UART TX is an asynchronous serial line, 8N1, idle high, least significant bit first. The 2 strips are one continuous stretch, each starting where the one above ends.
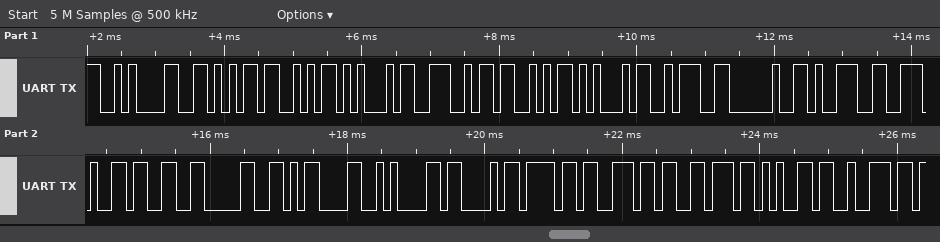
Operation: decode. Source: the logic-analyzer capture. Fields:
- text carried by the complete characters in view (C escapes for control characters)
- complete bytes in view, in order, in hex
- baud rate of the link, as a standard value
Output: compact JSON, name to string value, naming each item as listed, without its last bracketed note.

{"text carried by the complete characters in view": "\"\\nVSENSE: 9.30\\r\\nConver\"", "complete bytes in view, in order, in hex": "0x0A 0x56 0x53 0x45 0x4E 0x53 0x45 0x3A 0x20 0x39 0x2E 0x33 0x30 0x0D 0x0A 0x43 0x6F 0x6E 0x76 0x65 0x72", "baud rate of the link, as a standard value": "9600 baud"}
